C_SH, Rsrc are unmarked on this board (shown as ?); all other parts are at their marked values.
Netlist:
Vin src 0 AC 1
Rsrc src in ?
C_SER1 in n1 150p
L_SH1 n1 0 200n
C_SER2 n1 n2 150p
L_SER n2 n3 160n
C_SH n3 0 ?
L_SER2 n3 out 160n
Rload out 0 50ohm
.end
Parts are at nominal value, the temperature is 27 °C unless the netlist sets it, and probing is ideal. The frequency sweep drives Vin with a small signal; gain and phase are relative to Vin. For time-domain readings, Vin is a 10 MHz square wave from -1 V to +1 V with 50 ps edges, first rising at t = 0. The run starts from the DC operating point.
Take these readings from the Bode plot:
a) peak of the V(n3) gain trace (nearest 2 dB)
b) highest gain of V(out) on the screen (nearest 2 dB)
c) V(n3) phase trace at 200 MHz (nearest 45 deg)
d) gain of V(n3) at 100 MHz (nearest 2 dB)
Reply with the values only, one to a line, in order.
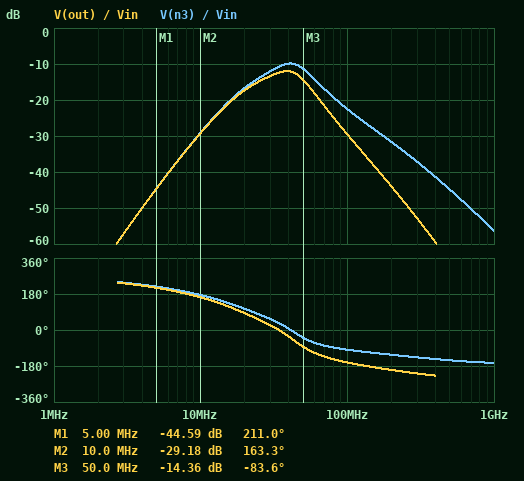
-10 dB
-12 dB
-135 deg
-22 dB
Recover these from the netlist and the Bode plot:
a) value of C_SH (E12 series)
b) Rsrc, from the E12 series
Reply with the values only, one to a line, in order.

100 pF
150 Ω
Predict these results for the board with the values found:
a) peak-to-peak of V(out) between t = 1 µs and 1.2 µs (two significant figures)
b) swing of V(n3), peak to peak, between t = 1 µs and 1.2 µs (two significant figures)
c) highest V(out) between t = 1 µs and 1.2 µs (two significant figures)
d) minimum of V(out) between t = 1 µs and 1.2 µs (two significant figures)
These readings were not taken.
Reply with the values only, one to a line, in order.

320 mV
390 mV
160 mV
-160 mV
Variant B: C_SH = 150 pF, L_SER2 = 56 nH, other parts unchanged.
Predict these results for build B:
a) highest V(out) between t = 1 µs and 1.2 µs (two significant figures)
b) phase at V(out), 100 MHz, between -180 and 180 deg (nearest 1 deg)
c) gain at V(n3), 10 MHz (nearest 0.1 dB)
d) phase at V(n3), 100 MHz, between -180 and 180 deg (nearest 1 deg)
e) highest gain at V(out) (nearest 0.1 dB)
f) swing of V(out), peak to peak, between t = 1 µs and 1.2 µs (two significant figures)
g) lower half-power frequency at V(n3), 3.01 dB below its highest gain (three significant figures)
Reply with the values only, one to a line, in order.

150 mV
-130 deg
-30.4 dB
-95 deg
-11.6 dB
300 mV
23.0 MHz
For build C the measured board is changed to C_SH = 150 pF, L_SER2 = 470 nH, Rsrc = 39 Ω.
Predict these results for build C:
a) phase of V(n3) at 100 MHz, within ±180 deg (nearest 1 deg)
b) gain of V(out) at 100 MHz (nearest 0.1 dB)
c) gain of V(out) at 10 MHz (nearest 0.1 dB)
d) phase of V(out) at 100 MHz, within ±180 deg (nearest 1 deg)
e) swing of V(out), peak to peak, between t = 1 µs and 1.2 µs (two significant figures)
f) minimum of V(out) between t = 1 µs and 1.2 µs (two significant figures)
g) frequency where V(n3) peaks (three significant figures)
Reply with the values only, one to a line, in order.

-134 deg
-33.7 dB
-23.6 dB
146 deg
560 mV
-280 mV
29.5 MHz
